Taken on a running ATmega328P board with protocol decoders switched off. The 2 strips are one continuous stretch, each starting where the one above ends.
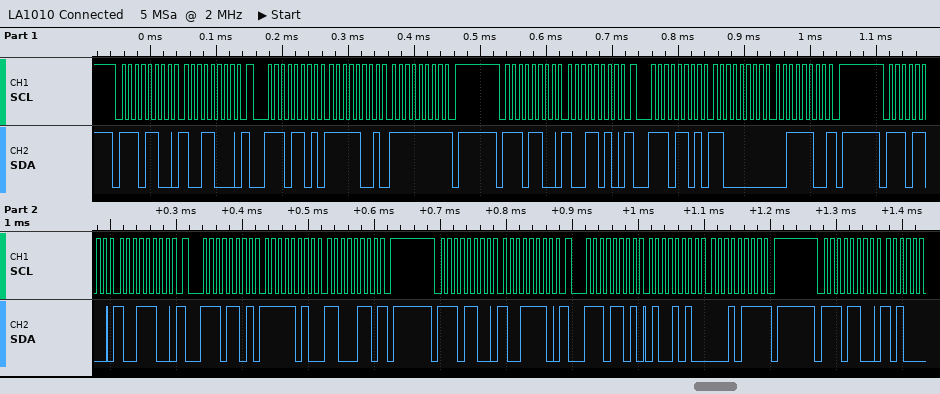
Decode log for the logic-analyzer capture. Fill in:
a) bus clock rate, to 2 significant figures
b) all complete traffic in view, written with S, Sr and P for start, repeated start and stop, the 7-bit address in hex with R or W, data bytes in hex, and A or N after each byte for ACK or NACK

100 kHz
S 76W A 98 A Sr 76R A F9 A FF N P S 76W A 9A A Sr 76R A C0 A 3C N P S 76W A 9C A Sr 76R A FA A C6 N P S 76W A 9E A Sr 76R A 4A A 17 N P S 76W A
